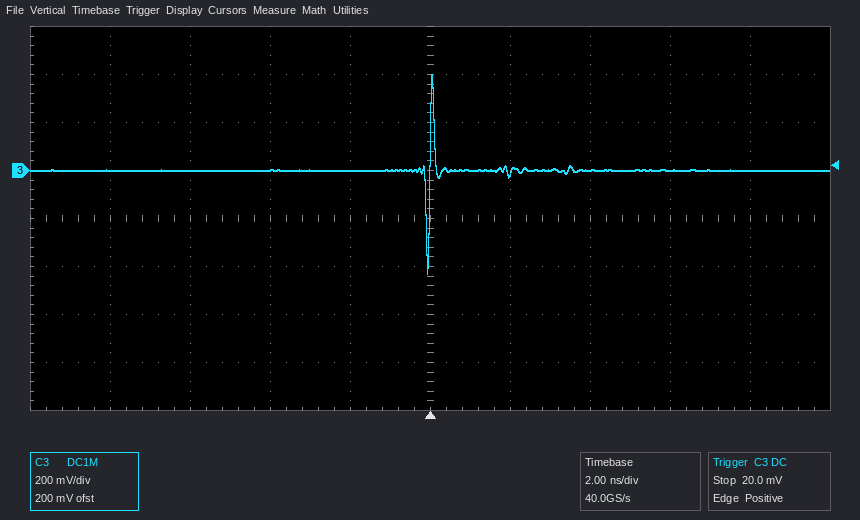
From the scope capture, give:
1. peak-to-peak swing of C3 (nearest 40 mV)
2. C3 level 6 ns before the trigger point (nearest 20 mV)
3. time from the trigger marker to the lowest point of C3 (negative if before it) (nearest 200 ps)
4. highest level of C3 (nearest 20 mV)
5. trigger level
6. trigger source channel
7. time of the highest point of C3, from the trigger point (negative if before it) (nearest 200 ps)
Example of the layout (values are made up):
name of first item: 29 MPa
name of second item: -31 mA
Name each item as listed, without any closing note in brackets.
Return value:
peak-to-peak swing of C3: 840 mV
C3 level 6 ns before the trigger point: 0 mV
time from the trigger marker to the lowest point of C3 (negative if before it): 0.0 ns
highest level of C3: 400 mV
trigger level: 20.0 mV
trigger source channel: C3
time of the highest point of C3, from the trigger point (negative if before it): 0.0 ns
